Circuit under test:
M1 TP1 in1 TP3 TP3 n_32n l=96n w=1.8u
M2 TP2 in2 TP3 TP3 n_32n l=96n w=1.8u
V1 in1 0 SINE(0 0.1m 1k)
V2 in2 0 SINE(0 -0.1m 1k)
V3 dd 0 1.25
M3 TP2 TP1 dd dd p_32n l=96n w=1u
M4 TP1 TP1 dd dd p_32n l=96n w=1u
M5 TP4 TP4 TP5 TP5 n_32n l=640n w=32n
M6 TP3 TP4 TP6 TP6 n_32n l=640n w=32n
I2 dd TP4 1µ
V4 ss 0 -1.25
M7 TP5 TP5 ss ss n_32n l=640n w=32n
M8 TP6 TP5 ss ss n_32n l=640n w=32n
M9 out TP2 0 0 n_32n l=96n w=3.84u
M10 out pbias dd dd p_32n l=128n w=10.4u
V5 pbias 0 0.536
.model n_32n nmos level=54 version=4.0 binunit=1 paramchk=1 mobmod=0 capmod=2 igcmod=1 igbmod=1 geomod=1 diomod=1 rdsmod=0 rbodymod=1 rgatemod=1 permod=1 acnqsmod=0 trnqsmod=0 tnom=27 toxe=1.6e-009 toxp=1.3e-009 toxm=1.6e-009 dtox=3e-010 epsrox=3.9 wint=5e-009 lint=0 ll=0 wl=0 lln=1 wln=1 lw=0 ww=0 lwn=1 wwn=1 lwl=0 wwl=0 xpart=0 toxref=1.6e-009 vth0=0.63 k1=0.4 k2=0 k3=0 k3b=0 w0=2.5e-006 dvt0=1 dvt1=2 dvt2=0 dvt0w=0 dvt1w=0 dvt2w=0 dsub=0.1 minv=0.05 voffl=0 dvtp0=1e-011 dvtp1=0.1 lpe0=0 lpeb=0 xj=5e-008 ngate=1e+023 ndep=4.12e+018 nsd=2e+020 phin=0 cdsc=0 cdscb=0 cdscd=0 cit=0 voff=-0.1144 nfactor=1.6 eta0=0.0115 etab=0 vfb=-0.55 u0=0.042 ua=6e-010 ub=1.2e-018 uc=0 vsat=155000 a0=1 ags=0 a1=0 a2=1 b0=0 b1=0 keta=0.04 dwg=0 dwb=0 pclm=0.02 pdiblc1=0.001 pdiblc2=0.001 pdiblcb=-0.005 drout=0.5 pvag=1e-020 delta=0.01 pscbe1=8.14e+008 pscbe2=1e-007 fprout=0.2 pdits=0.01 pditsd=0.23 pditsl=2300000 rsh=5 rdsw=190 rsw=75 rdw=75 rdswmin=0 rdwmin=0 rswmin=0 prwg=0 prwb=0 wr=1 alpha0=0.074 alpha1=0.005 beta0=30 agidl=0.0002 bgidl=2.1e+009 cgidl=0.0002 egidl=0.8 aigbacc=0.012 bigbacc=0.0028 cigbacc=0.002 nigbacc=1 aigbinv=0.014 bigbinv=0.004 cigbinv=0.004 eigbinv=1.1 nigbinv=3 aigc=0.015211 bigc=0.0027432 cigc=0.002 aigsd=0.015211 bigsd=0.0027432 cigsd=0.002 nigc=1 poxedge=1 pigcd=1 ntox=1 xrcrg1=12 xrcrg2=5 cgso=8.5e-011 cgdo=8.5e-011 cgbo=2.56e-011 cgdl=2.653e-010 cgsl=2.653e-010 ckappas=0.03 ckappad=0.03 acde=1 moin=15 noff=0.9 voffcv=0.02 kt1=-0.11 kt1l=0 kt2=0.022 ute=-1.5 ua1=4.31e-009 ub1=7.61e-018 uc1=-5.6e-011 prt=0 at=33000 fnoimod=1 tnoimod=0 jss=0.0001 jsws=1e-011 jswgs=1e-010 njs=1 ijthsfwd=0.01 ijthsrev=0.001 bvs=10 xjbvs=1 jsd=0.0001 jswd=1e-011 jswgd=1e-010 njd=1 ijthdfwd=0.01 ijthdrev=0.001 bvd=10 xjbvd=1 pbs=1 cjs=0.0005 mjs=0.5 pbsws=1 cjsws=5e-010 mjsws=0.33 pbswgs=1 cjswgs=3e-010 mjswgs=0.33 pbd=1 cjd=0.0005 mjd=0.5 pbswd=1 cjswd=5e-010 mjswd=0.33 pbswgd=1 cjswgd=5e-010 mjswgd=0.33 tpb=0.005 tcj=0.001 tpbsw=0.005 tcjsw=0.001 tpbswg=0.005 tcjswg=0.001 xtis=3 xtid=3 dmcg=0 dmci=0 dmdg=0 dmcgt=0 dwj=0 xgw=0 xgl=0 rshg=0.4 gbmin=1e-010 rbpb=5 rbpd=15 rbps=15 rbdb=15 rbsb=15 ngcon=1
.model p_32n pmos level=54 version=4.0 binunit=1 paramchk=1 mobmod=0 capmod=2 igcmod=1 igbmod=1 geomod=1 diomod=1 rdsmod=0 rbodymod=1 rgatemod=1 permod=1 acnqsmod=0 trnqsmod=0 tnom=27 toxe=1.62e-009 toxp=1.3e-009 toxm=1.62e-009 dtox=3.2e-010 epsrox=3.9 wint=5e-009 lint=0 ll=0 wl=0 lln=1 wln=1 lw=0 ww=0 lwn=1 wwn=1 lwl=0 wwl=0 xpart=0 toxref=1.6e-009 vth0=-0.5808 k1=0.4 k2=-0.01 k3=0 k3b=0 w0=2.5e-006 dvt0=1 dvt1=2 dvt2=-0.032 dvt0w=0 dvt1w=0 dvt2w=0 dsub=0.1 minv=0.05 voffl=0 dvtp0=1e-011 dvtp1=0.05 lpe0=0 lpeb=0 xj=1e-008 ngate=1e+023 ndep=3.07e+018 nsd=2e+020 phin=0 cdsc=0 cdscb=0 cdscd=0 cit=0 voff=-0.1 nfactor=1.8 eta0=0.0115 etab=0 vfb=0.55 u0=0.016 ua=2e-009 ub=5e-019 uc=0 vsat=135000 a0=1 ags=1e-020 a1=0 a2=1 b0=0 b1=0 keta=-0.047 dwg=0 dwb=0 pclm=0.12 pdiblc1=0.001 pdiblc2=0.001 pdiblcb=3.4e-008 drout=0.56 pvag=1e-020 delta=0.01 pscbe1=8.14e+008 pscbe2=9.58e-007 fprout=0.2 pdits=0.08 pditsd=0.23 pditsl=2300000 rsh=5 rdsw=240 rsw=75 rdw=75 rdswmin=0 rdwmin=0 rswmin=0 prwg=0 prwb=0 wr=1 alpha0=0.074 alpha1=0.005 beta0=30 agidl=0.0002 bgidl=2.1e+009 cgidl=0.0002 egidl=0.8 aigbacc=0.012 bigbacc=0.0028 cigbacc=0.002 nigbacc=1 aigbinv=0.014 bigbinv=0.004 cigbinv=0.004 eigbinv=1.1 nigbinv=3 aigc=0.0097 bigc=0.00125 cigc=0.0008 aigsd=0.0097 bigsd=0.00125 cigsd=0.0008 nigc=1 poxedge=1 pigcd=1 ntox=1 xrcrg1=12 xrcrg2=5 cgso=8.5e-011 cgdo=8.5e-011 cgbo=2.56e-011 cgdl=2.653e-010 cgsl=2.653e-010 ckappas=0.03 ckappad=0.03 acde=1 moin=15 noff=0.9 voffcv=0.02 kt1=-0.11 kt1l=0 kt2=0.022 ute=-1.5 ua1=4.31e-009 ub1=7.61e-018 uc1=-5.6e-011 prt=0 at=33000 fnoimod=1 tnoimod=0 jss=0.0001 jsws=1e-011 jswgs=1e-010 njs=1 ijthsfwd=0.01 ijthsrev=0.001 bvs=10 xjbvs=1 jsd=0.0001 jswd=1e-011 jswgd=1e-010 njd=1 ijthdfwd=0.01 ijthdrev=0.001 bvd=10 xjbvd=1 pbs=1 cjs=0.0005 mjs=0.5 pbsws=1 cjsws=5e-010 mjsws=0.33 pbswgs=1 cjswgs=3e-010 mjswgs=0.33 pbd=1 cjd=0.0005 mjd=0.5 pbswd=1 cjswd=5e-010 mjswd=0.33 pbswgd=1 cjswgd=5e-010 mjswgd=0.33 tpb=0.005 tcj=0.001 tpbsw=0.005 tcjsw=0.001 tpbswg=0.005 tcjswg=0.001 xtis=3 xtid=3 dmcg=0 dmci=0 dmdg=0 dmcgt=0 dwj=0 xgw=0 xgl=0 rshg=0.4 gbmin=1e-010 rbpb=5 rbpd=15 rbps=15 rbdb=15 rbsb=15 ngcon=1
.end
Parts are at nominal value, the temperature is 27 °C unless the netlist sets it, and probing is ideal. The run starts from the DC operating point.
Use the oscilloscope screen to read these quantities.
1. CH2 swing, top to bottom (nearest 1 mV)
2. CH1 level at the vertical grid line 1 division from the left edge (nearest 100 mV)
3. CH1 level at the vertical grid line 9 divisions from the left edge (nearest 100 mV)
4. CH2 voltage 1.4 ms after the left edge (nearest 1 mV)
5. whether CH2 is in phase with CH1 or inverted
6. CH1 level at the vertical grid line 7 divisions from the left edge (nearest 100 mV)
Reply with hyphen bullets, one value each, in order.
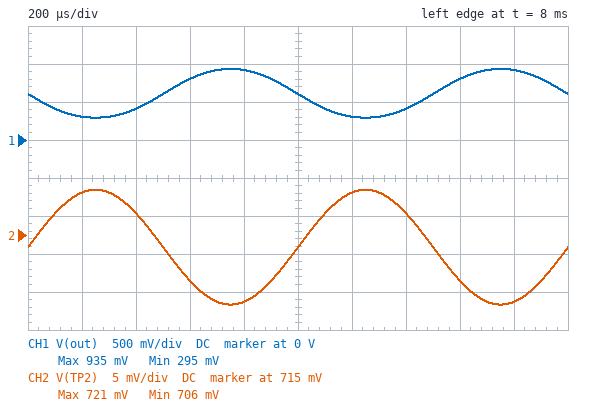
- 15 mV
- 300 mV
- 900 mV
- 718 mV
- inverted
- 400 mV
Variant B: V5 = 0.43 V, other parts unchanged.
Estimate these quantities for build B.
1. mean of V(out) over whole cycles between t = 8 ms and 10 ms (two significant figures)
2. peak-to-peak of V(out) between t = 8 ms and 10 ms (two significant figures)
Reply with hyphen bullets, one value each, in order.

- 1.2 V
- 14 mV
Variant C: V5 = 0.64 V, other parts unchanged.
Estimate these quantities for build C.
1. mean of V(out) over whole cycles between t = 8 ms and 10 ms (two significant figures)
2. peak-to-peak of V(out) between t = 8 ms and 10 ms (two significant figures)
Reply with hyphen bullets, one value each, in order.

- 18 mV
- 2.6 mV
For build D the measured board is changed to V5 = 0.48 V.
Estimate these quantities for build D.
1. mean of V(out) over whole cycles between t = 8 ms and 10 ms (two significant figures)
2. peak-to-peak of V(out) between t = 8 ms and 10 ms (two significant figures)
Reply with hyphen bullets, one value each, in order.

- 1.2 V
- 23 mV
